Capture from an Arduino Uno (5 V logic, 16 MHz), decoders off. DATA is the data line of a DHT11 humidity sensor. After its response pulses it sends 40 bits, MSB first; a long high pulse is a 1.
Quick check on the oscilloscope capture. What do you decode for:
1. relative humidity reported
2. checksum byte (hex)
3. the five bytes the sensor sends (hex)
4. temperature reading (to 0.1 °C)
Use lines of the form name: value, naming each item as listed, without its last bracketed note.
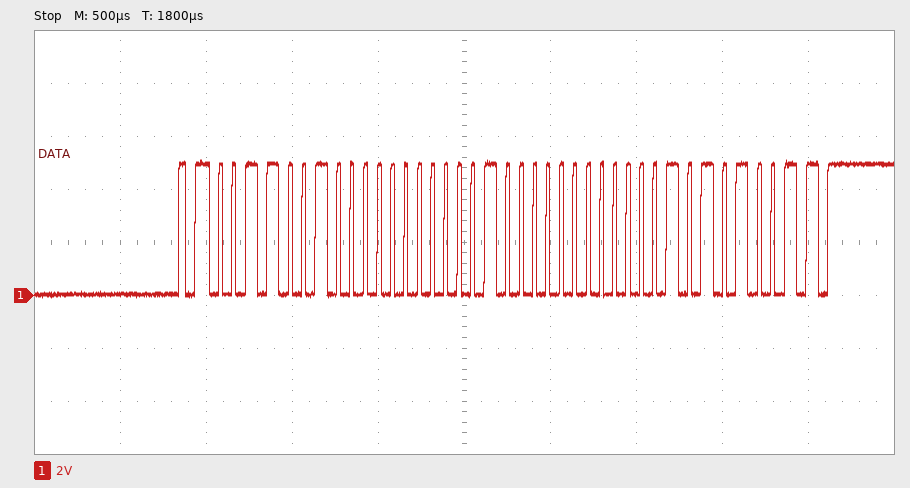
relative humidity reported: 50 %
checksum byte: 0x53
the five bytes the sensor sends: 32 00 20 01 53
temperature reading: 32.1 °C
